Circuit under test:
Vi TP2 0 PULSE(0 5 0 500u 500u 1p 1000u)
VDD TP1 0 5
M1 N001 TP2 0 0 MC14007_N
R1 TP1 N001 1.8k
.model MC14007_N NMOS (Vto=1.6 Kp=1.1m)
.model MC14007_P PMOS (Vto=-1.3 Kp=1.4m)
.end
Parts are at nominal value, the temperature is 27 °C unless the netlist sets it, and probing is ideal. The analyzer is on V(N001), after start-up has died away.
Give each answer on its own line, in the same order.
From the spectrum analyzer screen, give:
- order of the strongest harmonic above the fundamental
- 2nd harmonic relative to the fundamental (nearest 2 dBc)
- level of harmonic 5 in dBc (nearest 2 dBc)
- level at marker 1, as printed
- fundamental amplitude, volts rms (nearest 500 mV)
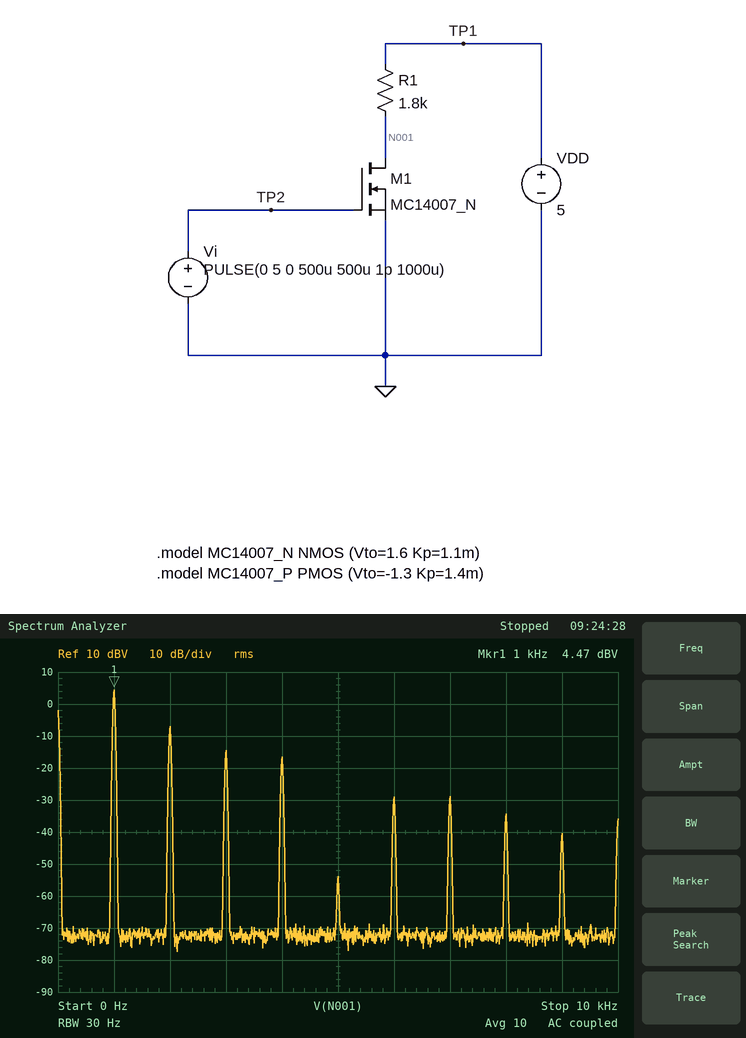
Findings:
2
-12 dBc
-58 dBc
4.47 dBV
1.5 V
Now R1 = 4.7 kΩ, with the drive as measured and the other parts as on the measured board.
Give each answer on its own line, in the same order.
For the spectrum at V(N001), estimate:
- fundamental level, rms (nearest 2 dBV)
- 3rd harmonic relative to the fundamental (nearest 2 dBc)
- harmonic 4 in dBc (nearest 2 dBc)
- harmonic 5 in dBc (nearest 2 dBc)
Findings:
6 dBV
-12 dBc
-48 dBc
-20 dBc
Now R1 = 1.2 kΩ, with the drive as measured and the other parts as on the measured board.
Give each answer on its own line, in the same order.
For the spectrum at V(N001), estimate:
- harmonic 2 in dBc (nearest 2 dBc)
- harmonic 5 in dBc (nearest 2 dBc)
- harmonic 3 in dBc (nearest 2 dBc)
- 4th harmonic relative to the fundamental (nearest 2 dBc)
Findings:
-8 dBc
-32 dBc
-38 dBc
-24 dBc
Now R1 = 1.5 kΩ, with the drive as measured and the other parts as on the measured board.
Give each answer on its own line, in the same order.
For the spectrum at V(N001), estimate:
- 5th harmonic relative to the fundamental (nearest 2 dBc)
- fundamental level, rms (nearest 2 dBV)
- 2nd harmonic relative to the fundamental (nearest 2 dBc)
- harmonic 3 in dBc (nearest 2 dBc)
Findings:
-36 dBc
4 dBV
-10 dBc
-24 dBc
